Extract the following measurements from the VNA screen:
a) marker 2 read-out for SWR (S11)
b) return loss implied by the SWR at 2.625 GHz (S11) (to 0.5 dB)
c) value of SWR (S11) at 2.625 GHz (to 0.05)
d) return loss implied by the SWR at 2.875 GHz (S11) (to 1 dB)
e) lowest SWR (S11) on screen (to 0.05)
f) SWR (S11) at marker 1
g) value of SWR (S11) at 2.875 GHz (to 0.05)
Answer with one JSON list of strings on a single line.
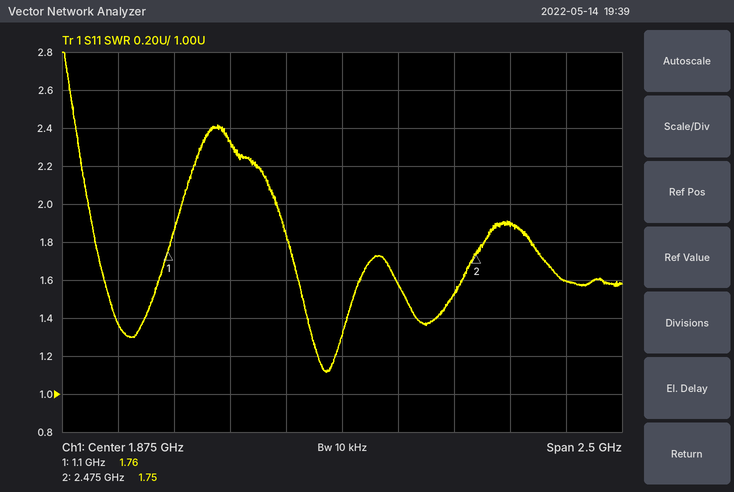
["1.75", "10.0 dB", "1.90", "13 dB", "1.10", "1.76", "1.60"]
